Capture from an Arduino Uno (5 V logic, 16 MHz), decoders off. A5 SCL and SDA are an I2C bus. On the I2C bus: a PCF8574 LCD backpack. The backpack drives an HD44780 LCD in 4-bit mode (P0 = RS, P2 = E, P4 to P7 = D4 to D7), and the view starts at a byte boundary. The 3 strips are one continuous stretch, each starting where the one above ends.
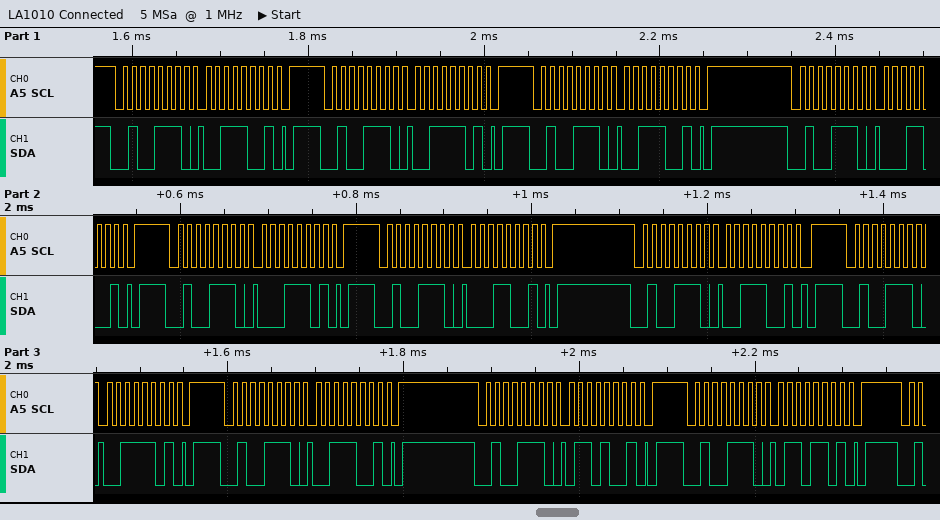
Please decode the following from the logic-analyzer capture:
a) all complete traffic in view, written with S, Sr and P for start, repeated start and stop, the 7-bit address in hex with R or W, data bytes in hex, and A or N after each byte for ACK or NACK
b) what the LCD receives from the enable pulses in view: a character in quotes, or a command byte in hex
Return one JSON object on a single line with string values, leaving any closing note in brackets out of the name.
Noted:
{"all complete traffic in view, written with S, Sr and P for start, repeated start and stop, the 7-bit address in hex with R or W, data bytes in hex, and A or N after each byte for ACK or NACK": "S 27W A 39 A P S 27W A 3D A P S 27W A 39 A P S 27W A 19 A P S 27W A 1D A P S 27W A 19 A P S 27W A 39 A P S 27W A 3D A P S 27W A 39 A P S 27W A 69 A P S 27W A 6D A P", "what the LCD receives from the enable pulses in view: a character in quotes, or a command byte in hex": "'1'"}
